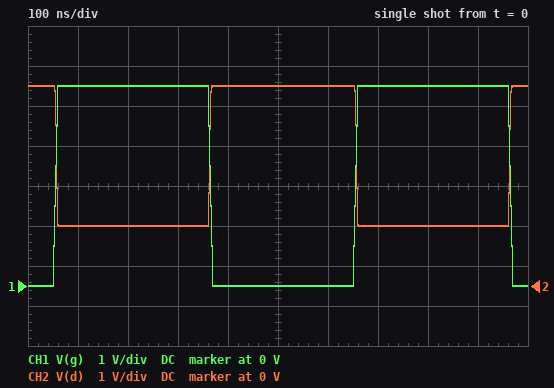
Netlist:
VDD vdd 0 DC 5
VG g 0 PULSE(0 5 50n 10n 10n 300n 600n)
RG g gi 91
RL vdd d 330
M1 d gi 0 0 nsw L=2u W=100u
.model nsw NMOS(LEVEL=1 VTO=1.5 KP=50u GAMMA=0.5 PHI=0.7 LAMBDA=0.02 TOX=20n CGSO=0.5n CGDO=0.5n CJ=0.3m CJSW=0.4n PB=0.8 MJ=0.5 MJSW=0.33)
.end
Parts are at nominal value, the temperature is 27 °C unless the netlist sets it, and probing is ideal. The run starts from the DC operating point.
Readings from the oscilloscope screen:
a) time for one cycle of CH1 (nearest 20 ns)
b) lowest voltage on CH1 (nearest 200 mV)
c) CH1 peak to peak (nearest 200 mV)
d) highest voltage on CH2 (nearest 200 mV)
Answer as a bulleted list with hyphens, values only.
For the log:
- 600 ns
- 0 V
- 5.0 V
- 5.0 V
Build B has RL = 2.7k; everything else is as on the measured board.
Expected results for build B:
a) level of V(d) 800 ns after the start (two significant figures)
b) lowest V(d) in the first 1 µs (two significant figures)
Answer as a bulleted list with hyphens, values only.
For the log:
- 210 mV
- 200 mV
